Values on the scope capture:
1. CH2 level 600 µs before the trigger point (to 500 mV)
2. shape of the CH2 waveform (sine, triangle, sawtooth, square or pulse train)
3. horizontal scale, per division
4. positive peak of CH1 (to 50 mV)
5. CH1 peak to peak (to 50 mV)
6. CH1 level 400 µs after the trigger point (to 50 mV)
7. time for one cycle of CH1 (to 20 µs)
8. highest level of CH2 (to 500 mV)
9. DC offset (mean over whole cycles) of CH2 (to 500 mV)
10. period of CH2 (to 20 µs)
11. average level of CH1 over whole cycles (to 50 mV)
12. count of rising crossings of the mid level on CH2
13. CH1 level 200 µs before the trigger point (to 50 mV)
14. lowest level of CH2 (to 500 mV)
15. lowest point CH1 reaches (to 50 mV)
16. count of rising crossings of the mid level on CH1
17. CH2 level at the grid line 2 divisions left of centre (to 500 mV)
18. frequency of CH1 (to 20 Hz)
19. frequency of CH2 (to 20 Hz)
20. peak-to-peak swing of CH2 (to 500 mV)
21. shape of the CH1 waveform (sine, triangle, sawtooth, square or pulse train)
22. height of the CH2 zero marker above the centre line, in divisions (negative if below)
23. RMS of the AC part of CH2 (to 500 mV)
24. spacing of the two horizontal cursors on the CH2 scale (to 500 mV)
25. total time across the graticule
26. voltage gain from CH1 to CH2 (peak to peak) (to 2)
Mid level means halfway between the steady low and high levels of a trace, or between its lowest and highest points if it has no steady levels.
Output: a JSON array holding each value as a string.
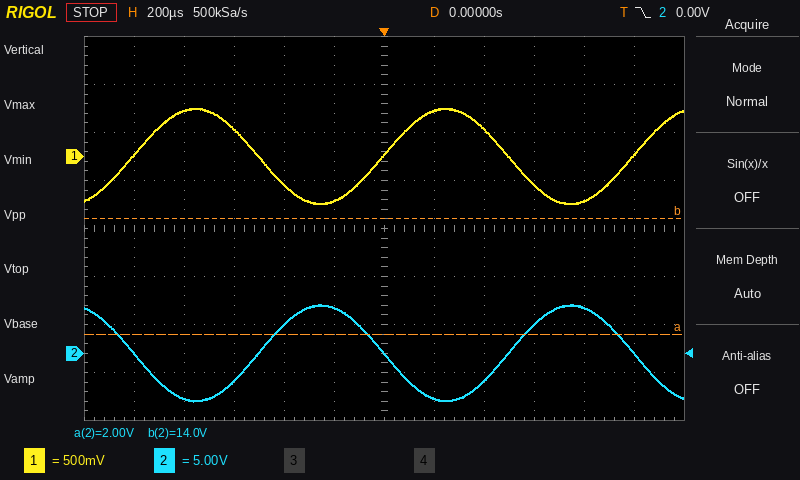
["-3.0 V", "sine", "200 µs", "500 mV", "1.00 V", "300 mV", "1.00 ms", "5.0 V", "0.0 V", "1.00 ms", "0 mV", "2", "-450 mV", "-5.0 V", "-500 mV", "3", "3.0 V", "1.00 kHz", "1.00 kHz", "10.0 V", "sine", "-2.6 div", "3.5 V", "12.0 V", "2.4 ms", "10"]
